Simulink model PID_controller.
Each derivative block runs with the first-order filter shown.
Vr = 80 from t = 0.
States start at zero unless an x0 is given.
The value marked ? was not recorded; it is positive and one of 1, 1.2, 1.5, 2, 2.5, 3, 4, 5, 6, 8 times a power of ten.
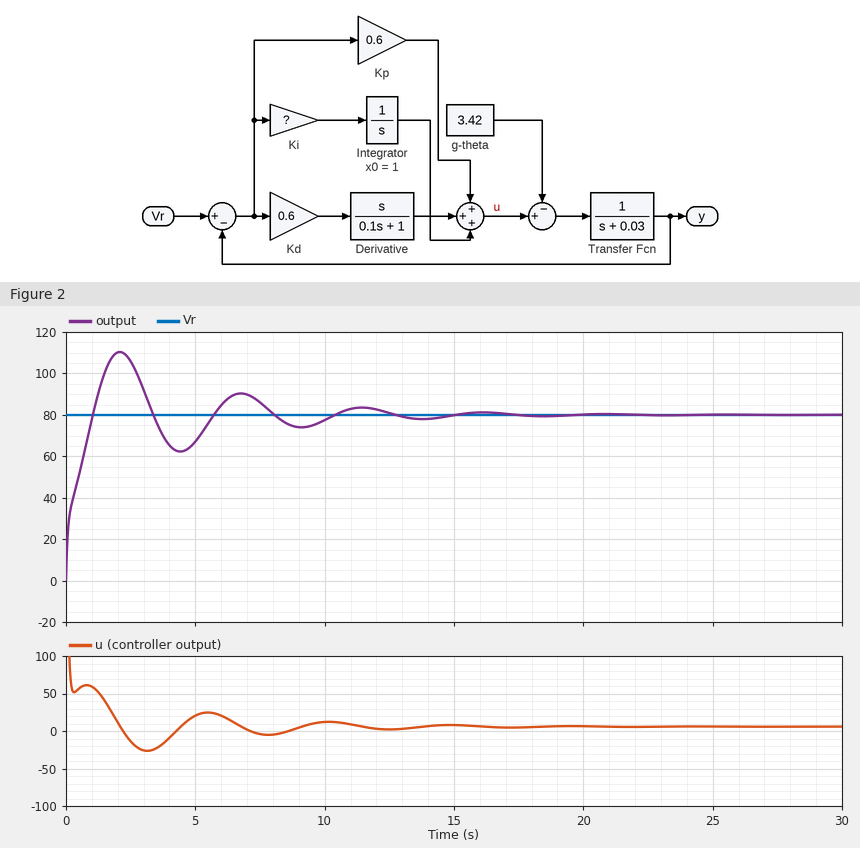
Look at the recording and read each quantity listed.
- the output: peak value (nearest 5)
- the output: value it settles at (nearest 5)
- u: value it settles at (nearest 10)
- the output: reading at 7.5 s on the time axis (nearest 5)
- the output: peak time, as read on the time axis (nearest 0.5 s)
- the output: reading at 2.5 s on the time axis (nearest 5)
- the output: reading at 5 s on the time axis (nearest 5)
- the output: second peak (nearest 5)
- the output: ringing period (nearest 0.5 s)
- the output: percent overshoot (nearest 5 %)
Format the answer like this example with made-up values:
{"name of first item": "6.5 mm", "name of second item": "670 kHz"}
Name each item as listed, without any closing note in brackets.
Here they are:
{"the output: peak value": "110", "the output: value it settles at": "80", "u: value it settles at": "10", "the output: reading at 7.5 s on the time axis": "85", "the output: peak time, as read on the time axis": "2.0 s", "the output: reading at 2.5 s on the time axis": "105", "the output: reading at 5 s on the time axis": "65", "the output: second peak": "90", "the output: ringing period": "4.5 s", "the output: percent overshoot": "40 %"}
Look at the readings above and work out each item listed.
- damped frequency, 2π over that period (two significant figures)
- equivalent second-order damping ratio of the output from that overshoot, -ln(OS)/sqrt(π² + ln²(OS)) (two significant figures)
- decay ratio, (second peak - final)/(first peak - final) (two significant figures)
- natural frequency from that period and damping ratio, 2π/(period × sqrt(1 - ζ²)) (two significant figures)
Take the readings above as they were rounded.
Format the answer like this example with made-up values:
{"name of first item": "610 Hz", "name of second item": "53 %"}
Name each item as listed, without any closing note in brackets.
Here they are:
{"damped frequency, 2π over that period": "1.4 rad/s", "equivalent second-order damping ratio of the output from that overshoot, -ln(OS)/sqrt(π² + ln²(OS))": "0.28", "decay ratio, (second peak - final)/(first peak - final)": "0.33", "natural frequency from that period and damping ratio, 2π/(period × sqrt(1 - ζ²))": "1.5 rad/s"}
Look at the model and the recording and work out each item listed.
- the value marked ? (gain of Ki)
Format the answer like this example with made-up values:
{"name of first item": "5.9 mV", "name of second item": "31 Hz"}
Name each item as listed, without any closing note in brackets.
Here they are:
{"the value marked ?": "3"}
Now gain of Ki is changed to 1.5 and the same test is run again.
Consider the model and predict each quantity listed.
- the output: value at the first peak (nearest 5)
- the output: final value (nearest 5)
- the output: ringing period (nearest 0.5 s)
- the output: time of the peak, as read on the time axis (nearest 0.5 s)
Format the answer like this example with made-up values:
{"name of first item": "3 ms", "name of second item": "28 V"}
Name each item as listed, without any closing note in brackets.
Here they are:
{"the output: value at the first peak": "105", "the output: final value": "80", "the output: ringing period": "6.5 s", "the output: time of the peak, as read on the time axis": "3.0 s"}
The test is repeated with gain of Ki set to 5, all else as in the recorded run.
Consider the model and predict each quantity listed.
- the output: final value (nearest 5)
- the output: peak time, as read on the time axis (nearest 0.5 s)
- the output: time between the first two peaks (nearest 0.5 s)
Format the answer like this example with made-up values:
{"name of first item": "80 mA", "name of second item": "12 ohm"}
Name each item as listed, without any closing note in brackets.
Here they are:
{"the output: final value": "80", "the output: peak time, as read on the time axis": "1.5 s", "the output: time between the first two peaks": "3.5 s"}
